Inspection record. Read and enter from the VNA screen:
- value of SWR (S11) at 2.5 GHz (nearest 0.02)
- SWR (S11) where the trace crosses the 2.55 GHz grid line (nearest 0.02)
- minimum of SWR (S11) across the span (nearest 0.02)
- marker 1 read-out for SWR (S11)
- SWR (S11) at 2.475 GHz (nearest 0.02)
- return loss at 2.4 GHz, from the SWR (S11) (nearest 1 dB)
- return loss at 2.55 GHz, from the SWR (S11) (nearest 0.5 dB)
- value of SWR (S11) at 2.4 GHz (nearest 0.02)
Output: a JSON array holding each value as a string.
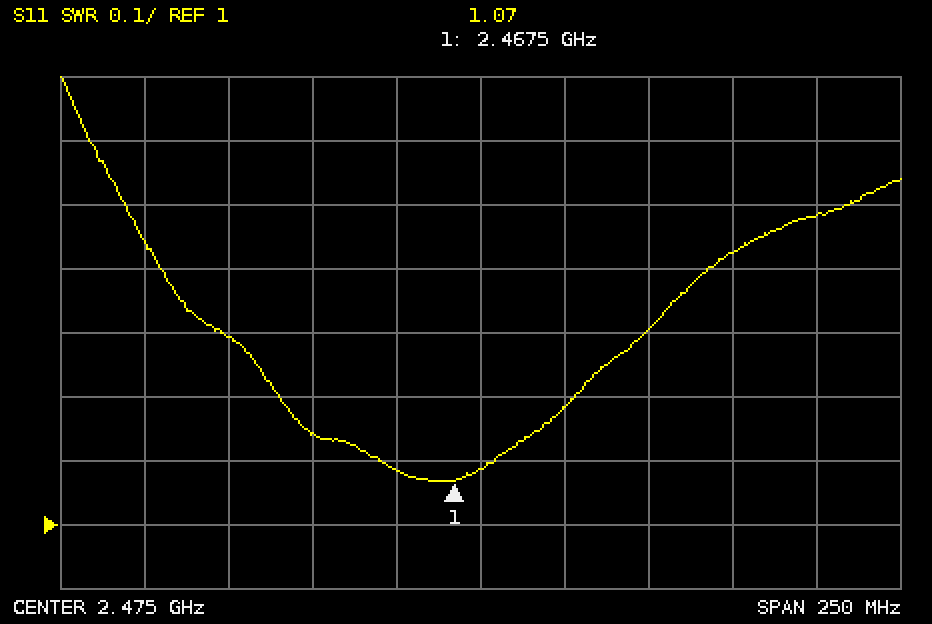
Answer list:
["1.18", "1.42", "1.06", "1.07", "1.08", "18 dB", "15.0 dB", "1.30"]
